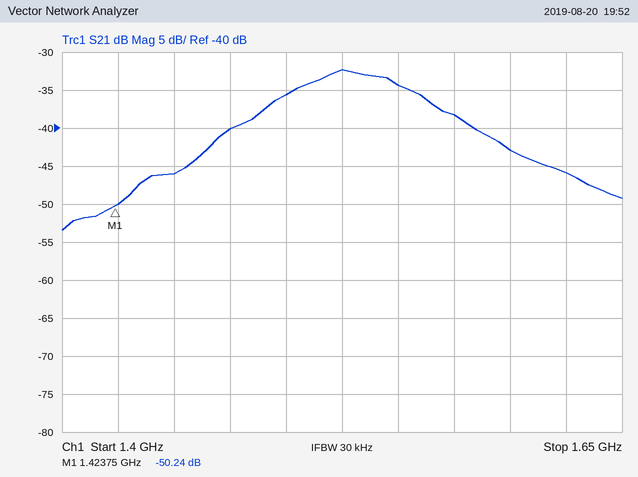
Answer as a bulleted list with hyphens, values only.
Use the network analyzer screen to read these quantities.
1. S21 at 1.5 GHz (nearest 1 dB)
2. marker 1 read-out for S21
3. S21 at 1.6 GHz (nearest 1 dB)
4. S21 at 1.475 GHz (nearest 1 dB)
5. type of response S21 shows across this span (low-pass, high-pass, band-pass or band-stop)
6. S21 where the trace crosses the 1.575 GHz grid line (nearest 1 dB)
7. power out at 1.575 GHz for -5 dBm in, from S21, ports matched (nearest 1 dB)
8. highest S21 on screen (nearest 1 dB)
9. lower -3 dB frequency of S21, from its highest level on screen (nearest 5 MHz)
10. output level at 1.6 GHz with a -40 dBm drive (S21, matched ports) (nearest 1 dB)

- -36 dB
- -50.24 dB
- -43 dB
- -40 dB
- band-pass
- -38 dB
- -43 dBm
- -32 dB
- 1.500 GHz
- -83 dBm
